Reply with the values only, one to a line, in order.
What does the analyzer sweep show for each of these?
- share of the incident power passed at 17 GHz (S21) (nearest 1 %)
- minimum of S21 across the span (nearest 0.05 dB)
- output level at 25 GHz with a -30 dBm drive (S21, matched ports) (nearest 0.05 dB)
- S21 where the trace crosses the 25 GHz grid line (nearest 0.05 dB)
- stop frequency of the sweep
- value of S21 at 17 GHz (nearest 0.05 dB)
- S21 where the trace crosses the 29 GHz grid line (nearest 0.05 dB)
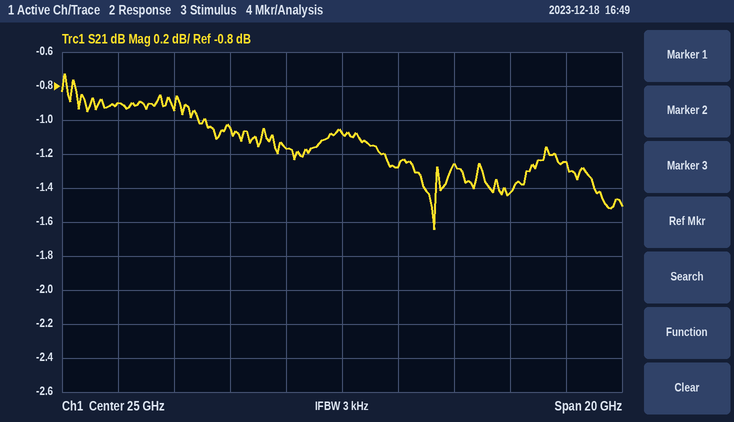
81 %
-1.65 dB
-31.10 dBm
-1.10 dB
35 GHz
-0.90 dB
-1.25 dB
